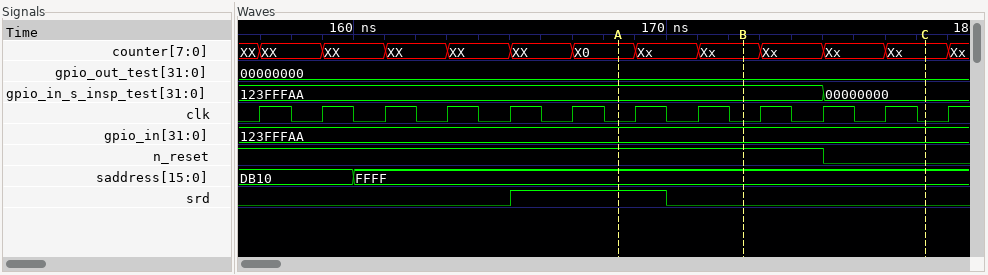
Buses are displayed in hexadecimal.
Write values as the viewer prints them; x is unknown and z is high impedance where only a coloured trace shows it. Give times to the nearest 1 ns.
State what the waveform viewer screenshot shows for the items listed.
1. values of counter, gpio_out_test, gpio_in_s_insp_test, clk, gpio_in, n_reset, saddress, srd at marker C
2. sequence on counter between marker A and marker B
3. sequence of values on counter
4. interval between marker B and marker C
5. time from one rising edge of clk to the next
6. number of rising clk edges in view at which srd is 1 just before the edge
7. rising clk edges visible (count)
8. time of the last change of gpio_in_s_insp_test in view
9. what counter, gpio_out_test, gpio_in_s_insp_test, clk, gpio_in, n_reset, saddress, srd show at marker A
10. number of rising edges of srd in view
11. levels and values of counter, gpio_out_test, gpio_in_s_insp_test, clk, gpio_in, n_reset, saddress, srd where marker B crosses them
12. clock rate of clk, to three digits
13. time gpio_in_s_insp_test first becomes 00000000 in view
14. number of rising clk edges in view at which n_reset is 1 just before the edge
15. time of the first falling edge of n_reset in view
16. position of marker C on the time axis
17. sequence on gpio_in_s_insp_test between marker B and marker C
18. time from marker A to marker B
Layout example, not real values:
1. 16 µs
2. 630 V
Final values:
1. counter=Xx, gpio_out_test=00000000, gpio_in_s_insp_test=00000000, clk=0, gpio_in=123FFFAA, n_reset=0, saddress=FFFF, srd=0
2. X0, Xx, Xx
3. XX, XX, XX, XX, XX, XX, X0, Xx, Xx, Xx, Xx, Xx, Xx
4. 6 ns
5. 2 ns
6. 2
7. 12
8. 175 ns
9. counter=X0, gpio_out_test=00000000, gpio_in_s_insp_test=123FFFAA, clk=0, gpio_in=123FFFAA, n_reset=1, saddress=FFFF, srd=1
10. 1
11. counter=Xx, gpio_out_test=00000000, gpio_in_s_insp_test=123FFFAA, clk=0, gpio_in=123FFFAA, n_reset=1, saddress=FFFF, srd=0
12. 500 MHz
13. 175 ns
14. 10
15. 175 ns
16. 178 ns
17. 123FFFAA, 00000000
18. 4 ns
